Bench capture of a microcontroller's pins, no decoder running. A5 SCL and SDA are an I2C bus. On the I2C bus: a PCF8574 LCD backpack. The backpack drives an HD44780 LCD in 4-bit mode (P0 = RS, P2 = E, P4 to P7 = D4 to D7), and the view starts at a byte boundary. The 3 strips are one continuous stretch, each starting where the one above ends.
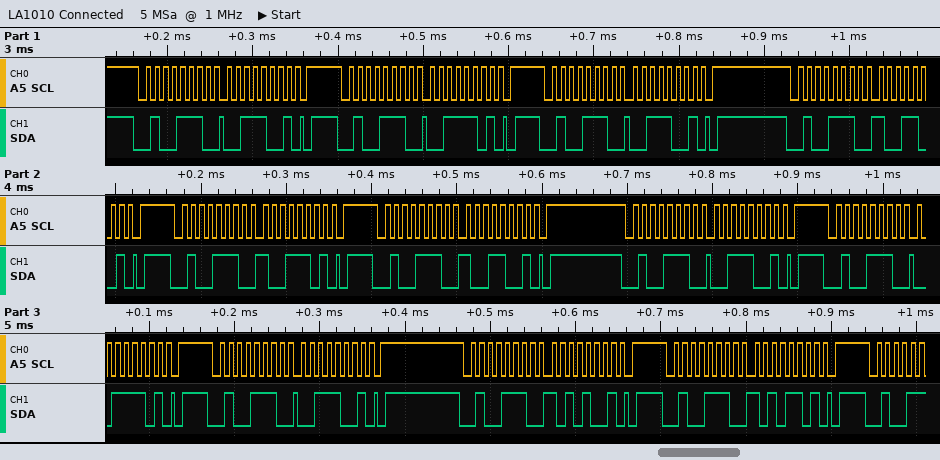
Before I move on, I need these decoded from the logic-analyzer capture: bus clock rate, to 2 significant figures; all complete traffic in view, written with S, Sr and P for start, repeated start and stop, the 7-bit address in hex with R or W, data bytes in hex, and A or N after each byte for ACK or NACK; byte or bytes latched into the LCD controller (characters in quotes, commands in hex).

100 kHz
S 27W A 39 A P S 27W A 3D A P S 27W A 39 A P S 27W A 99 A P S 27W A 9D A P S 27W A 99 A P S 27W A 39 A P S 27W A 3D A P S 27W A 39 A P S 27W A A9 A P S 27W A AD A P
'9'
